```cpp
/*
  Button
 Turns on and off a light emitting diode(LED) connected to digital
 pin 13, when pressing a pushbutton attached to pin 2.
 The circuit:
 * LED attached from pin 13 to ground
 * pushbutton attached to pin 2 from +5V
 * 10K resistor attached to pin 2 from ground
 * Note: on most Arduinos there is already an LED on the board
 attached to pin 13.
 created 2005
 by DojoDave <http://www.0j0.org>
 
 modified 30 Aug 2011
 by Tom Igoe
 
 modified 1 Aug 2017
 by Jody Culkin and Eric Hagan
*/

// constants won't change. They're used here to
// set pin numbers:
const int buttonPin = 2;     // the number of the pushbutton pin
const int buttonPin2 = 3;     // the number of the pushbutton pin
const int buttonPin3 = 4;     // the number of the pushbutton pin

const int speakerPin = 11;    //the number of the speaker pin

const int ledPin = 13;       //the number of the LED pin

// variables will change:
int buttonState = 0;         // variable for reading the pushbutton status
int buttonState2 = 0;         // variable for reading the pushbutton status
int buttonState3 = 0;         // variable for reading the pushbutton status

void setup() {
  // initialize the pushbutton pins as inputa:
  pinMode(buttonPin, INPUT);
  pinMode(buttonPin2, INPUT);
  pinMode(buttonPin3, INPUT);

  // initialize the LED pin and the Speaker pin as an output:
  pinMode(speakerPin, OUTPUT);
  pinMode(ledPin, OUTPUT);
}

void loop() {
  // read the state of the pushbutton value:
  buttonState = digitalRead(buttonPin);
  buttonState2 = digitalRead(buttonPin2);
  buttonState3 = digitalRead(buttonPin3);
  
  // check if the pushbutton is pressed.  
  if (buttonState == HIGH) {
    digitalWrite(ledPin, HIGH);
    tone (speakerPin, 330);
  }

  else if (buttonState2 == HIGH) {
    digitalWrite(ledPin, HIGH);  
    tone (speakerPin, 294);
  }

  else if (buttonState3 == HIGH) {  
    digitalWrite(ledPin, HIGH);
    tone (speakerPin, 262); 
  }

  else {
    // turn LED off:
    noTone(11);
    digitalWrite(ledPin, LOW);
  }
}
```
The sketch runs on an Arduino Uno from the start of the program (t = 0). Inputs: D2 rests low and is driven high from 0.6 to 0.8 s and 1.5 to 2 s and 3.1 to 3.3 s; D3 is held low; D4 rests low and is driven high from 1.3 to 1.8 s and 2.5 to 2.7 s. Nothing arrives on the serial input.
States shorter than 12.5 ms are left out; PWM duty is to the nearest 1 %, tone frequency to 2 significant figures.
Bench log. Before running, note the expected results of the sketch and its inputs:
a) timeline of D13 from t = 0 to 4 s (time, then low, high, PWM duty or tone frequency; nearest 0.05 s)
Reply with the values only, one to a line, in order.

0 s low; 0.6 s high; 0.8 s low; 1.3 s high; 2 s low; 2.5 s high; 2.7 s low; 3.1 s high; 3.3 s low
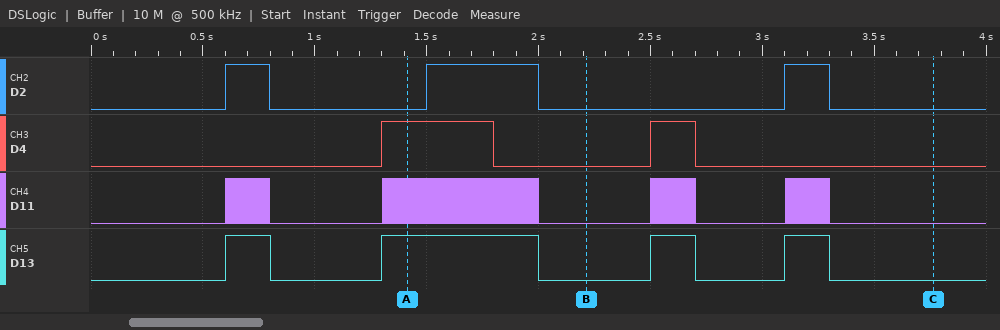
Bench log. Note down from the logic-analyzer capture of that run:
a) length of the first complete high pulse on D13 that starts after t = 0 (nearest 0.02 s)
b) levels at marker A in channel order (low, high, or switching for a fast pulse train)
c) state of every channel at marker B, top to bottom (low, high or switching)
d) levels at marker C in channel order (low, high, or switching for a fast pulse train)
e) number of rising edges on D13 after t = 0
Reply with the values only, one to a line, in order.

0.20 s
D2 low, D4 high, D11 switching, D13 high
D2 low, D4 low, D11 low, D13 low
D2 low, D4 low, D11 low, D13 low
4
